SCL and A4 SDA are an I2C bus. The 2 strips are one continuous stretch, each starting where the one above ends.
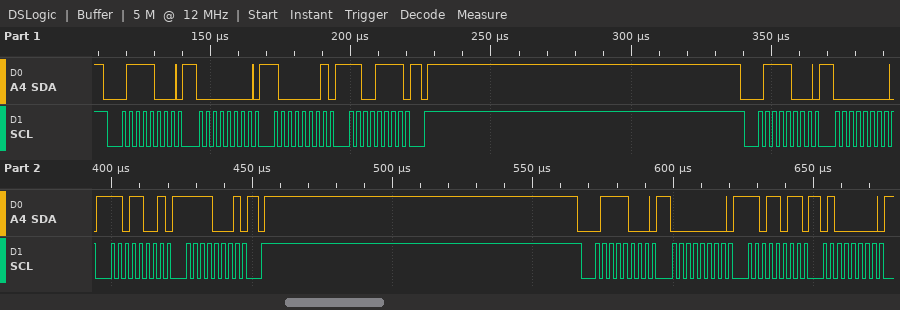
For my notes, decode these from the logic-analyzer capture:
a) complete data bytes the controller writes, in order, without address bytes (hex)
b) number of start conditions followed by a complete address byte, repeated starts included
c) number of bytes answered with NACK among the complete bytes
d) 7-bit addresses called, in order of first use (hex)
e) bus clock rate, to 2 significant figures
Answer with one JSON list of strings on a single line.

["00 81 CF 00 D9 F1 00 DB 40", "3", "0", "0x3C", "400 kHz"]
